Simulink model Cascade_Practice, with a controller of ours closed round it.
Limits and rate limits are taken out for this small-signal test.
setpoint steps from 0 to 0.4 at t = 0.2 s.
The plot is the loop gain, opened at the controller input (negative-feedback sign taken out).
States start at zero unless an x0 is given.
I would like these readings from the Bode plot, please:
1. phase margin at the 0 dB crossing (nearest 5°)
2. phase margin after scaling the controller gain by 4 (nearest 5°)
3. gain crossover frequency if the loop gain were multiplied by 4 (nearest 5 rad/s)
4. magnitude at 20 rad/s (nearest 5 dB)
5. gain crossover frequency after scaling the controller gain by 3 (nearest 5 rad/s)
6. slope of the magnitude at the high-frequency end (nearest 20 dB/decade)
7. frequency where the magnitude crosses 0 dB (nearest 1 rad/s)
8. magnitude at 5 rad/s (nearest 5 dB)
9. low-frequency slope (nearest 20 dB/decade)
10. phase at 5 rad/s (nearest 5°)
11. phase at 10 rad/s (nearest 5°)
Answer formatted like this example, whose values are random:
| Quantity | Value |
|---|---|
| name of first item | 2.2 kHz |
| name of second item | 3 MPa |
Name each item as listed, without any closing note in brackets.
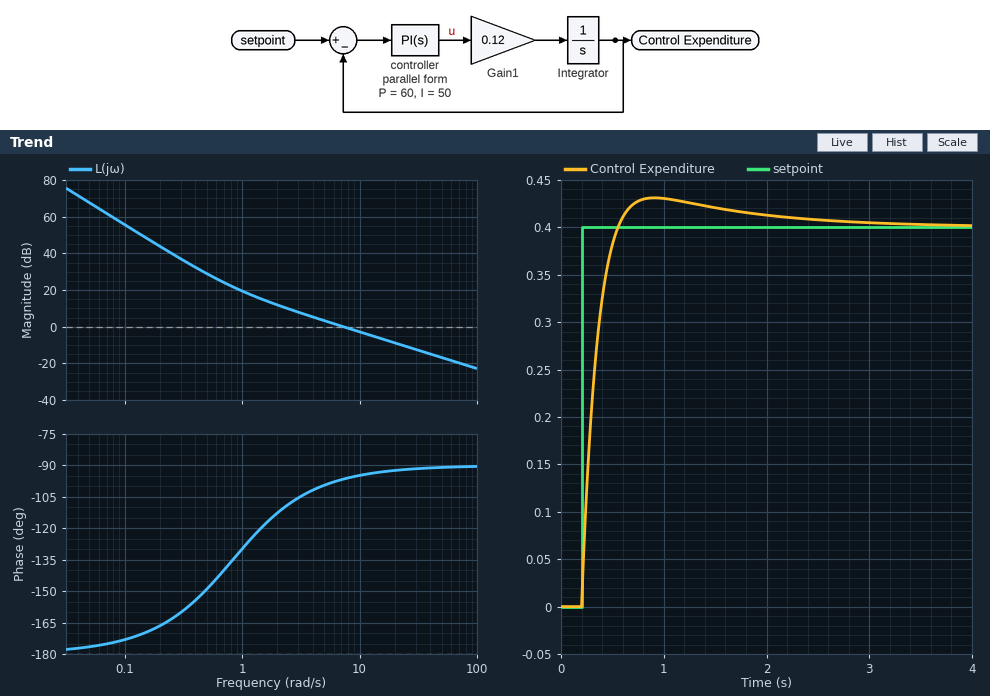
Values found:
| Quantity | Value |
|---|---|
| phase margin at the 0 dB crossing | 85° |
| phase margin after scaling the controller gain by 4 | 90° |
| gain crossover frequency if the loop gain were multiplied by 4 | 30 rad/s |
| magnitude at 20 rad/s | -10 dB |
| gain crossover frequency after scaling the controller gain by 3 | 20 rad/s |
| slope of the magnitude at the high-frequency end | -20 dB/decade |
| frequency where the magnitude crosses 0 dB | 7 rad/s |
| magnitude at 5 rad/s | 5 dB |
| low-frequency slope | -40 dB/decade |
| phase at 5 rad/s | -100° |
| phase at 10 rad/s | -95° |
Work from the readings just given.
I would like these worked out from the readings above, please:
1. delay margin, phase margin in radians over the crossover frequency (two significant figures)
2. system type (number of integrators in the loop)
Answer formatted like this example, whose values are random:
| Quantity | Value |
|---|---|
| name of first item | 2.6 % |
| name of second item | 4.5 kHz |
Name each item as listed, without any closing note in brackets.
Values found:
| Quantity | Value |
|---|---|
| delay margin, phase margin in radians over the crossover frequency | 0.21 s |
| system type | 2 |
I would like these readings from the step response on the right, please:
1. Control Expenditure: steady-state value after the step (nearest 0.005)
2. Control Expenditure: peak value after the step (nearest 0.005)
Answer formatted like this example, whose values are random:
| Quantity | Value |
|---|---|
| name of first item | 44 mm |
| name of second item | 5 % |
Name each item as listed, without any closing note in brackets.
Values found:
| Quantity | Value |
|---|---|
| Control Expenditure: steady-state value after the step | 0.400 |
| Control Expenditure: peak value after the step | 0.430 |
